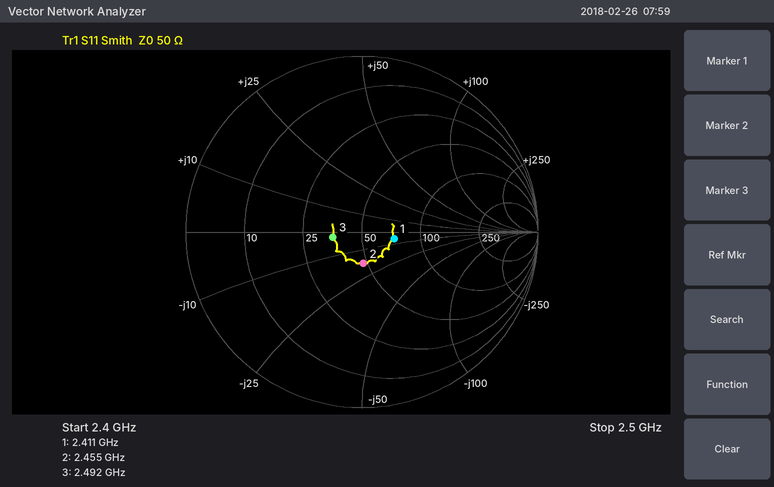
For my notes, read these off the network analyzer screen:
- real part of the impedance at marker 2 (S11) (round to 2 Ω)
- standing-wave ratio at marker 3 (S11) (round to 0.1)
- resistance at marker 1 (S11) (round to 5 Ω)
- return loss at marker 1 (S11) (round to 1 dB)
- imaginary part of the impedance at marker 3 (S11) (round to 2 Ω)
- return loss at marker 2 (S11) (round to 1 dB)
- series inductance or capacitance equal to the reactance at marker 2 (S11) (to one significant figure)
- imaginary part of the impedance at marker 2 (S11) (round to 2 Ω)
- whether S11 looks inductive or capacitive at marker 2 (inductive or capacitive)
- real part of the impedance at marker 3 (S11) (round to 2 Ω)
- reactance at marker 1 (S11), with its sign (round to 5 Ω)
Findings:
48 Ω
1.4
70 Ω
15 dB
-2 Ω
15 dB
4 pF
-18 Ω
capacitive
36 Ω
-5 Ω
